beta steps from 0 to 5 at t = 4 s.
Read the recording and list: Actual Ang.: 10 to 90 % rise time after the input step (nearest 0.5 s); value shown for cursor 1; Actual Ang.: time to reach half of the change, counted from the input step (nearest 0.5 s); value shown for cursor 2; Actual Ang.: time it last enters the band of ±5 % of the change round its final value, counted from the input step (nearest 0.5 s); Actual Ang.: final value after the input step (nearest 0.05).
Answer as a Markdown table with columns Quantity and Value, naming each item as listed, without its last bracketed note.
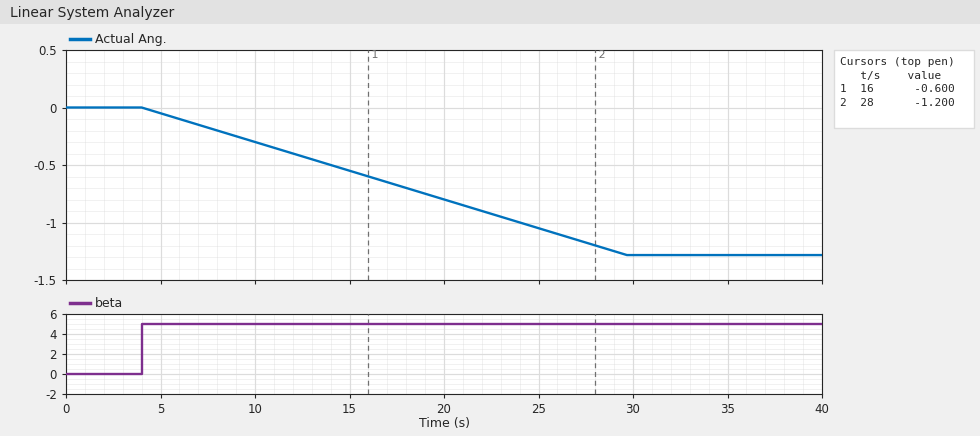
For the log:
| Quantity | Value |
|---|---|
| Actual Ang.: 10 to 90 % rise time after the input step | 20.5 s |
| value shown for cursor 1 | -0.600 |
| Actual Ang.: time to reach half of the change, counted from the input step | 13.0 s |
| value shown for cursor 2 | -1.200 |
| Actual Ang.: time it last enters the band of ±5 % of the change round its final value, counted from the input step | 24.5 s |
| Actual Ang.: final value after the input step | -1.30 |
